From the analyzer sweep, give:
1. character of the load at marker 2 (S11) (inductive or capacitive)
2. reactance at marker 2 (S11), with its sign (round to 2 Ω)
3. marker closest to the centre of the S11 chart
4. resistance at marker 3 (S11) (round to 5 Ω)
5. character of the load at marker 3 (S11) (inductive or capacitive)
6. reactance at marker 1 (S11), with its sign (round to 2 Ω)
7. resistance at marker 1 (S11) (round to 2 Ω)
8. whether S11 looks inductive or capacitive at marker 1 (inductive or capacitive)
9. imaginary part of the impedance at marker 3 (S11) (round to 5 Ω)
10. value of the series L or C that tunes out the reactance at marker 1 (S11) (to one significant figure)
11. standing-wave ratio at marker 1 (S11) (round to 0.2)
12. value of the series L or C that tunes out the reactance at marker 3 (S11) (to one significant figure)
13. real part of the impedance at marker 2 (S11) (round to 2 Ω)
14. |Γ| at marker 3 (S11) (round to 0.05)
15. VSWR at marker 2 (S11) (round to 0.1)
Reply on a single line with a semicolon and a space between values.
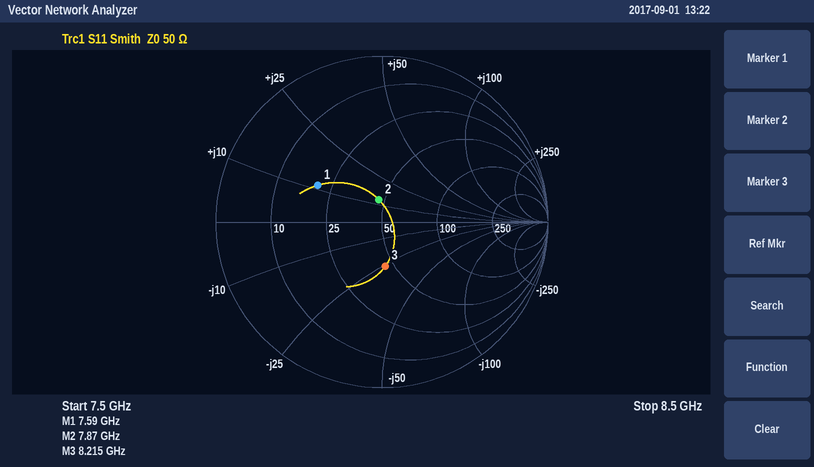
inductive; +12 Ω; marker 2; 45 Ω; capacitive; +12 Ω; 20 Ω; inductive; -25 Ω; 2 pF; 2.6; 500 pH; 46 Ω; 0.25; 1.3
